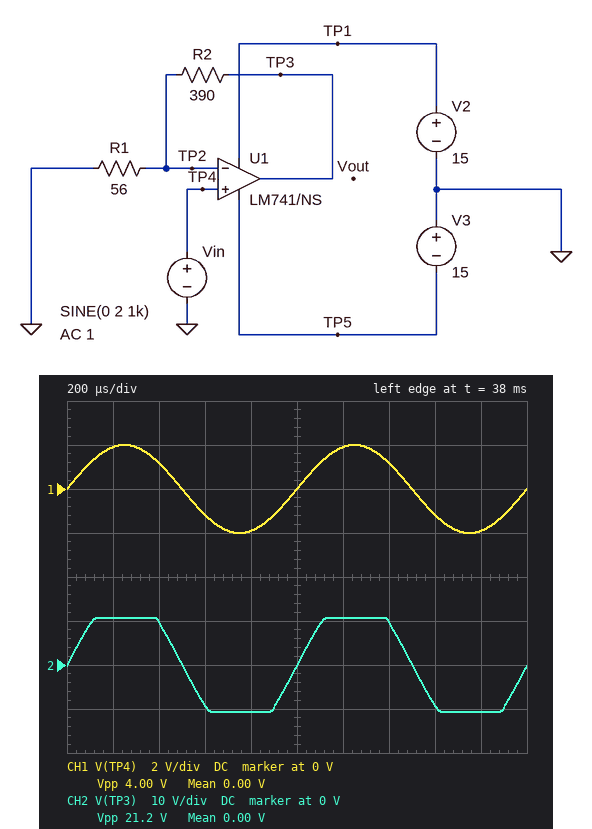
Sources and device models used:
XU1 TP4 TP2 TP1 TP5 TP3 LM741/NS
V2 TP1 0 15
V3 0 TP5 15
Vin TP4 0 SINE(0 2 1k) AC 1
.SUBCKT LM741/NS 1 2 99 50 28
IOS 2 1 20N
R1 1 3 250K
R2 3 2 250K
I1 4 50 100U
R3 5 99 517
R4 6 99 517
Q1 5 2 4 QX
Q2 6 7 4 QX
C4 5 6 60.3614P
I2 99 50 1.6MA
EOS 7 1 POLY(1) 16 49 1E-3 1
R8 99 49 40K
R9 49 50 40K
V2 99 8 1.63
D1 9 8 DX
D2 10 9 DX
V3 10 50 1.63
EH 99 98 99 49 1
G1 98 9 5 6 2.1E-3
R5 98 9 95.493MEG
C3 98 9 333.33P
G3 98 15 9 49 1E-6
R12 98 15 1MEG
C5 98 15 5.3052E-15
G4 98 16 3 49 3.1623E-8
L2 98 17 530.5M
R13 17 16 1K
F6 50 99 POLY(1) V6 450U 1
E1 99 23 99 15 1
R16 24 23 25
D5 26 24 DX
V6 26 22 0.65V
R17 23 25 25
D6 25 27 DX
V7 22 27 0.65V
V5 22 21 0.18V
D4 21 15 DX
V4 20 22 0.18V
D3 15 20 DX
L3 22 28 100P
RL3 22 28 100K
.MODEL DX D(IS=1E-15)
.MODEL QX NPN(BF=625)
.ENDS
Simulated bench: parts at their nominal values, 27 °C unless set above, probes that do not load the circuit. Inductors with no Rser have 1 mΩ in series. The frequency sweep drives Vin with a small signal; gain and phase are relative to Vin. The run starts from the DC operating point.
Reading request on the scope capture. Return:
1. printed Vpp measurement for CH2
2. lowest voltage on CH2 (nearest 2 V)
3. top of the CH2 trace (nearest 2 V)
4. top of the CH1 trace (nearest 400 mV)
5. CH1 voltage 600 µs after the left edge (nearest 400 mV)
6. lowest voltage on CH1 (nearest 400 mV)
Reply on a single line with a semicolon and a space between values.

21.2 V; -10 V; 10 V; 2.0 V; -1.2 V; -2.0 V
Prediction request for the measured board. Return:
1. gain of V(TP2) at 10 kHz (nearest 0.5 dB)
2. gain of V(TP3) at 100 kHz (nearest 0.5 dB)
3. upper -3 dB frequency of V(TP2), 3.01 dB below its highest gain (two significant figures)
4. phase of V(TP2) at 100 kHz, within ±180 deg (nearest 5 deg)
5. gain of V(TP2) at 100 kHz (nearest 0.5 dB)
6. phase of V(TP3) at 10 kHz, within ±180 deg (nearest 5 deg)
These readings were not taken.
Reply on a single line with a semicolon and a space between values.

0 dB; 14.5 dB; 93 kHz; -50 deg; -3.5 dB; -5 deg
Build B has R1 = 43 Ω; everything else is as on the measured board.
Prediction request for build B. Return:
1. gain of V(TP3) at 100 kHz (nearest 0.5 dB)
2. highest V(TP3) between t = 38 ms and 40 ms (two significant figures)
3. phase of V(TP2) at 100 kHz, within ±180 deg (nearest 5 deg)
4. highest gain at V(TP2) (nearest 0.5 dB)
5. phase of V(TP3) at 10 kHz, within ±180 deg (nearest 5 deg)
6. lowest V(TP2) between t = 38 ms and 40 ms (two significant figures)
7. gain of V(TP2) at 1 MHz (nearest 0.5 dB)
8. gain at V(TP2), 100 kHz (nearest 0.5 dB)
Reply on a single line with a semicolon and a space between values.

15.5 dB; 10 V; -55 deg; 0 dB; -10 deg; -1.0 V; -23.5 dB; -4.5 dB
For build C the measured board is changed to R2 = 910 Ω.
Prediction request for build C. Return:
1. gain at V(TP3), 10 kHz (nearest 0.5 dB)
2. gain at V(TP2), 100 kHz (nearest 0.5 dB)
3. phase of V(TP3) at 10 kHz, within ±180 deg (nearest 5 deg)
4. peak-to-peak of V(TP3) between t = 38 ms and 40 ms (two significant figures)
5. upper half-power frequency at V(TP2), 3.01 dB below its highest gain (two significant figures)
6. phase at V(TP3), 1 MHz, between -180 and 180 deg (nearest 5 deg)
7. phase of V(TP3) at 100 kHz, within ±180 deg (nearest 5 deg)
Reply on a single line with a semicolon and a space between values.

24.5 dB; -7.0 dB; -10 deg; 27 V; 50 kHz; -110 deg; -65 deg
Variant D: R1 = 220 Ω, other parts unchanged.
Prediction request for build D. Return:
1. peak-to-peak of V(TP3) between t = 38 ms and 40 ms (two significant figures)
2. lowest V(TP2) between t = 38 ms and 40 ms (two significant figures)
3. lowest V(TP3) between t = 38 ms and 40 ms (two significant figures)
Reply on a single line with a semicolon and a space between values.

11 V; -2.0 V; -5.5 V
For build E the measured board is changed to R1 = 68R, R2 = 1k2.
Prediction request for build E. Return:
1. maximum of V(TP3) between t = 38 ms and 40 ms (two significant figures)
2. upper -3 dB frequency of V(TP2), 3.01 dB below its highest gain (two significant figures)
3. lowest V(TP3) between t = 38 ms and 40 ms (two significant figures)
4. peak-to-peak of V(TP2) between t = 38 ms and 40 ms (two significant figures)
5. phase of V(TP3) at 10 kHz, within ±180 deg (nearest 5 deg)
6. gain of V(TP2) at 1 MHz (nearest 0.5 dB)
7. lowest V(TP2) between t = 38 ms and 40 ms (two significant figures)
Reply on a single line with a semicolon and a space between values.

14 V; 48 kHz; -14 V; 1.5 V; -10 deg; -27.0 dB; -730 mV
